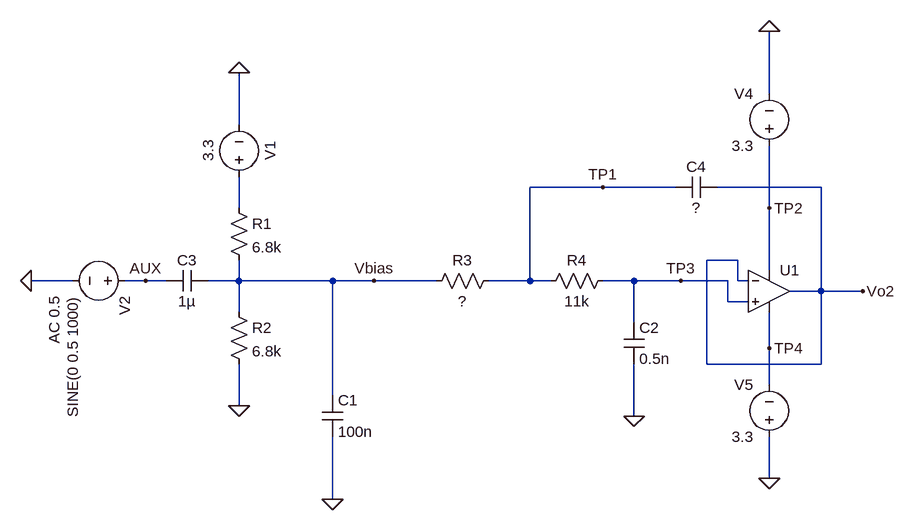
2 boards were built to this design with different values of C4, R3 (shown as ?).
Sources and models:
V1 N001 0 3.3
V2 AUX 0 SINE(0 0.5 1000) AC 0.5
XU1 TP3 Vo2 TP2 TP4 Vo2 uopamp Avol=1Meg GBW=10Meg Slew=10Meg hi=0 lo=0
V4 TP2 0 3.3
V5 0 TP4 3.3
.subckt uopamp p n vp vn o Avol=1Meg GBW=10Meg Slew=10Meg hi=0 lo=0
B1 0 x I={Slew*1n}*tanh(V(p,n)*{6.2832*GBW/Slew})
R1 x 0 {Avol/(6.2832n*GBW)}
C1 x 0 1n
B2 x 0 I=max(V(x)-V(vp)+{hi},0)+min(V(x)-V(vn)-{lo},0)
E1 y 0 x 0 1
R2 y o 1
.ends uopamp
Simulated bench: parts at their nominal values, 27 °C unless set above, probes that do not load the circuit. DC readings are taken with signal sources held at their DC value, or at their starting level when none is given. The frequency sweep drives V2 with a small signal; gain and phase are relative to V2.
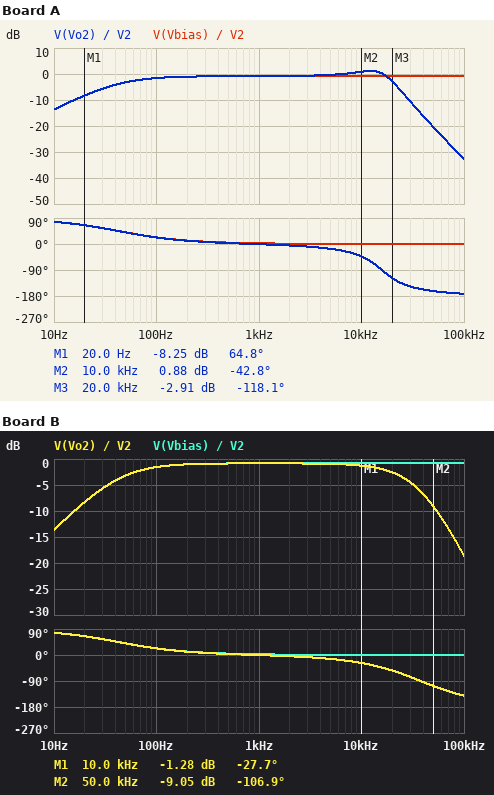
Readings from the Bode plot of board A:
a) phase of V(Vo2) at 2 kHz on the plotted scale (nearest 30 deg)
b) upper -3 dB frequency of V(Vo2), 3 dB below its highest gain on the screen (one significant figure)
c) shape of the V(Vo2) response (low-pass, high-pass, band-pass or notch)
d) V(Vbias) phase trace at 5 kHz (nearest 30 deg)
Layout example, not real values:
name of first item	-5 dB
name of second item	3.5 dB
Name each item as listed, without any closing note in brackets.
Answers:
phase of V(Vo2) at 2 kHz on the plotted scale	0 deg
upper -3 dB frequency of V(Vo2), 3 dB below its highest gain on the screen	20 kHz
shape of the V(Vo2) response	band-pass
V(Vbias) phase trace at 5 kHz	0 deg
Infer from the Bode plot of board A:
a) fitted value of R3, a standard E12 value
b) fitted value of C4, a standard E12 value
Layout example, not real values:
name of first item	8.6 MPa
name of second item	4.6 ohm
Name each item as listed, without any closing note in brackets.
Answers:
fitted value of R3, a standard E12 value	6.8 kΩ
fitted value of C4, a standard E12 value	2.7 nF
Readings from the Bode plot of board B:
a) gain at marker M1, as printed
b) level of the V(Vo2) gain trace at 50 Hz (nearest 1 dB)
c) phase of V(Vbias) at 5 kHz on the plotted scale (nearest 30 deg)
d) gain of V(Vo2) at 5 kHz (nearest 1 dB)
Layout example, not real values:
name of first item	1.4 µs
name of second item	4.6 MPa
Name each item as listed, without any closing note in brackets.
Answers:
gain at marker M1, as printed	-1.28 dB
level of the V(Vo2) gain trace at 50 Hz	-3 dB
phase of V(Vbias) at 5 kHz on the plotted scale	0 deg
gain of V(Vo2) at 5 kHz	-1 dB
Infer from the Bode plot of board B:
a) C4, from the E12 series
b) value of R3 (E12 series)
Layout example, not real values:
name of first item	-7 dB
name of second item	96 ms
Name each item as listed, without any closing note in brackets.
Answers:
C4, from the E12 series	680 pF
value of R3	4.7 kΩ
